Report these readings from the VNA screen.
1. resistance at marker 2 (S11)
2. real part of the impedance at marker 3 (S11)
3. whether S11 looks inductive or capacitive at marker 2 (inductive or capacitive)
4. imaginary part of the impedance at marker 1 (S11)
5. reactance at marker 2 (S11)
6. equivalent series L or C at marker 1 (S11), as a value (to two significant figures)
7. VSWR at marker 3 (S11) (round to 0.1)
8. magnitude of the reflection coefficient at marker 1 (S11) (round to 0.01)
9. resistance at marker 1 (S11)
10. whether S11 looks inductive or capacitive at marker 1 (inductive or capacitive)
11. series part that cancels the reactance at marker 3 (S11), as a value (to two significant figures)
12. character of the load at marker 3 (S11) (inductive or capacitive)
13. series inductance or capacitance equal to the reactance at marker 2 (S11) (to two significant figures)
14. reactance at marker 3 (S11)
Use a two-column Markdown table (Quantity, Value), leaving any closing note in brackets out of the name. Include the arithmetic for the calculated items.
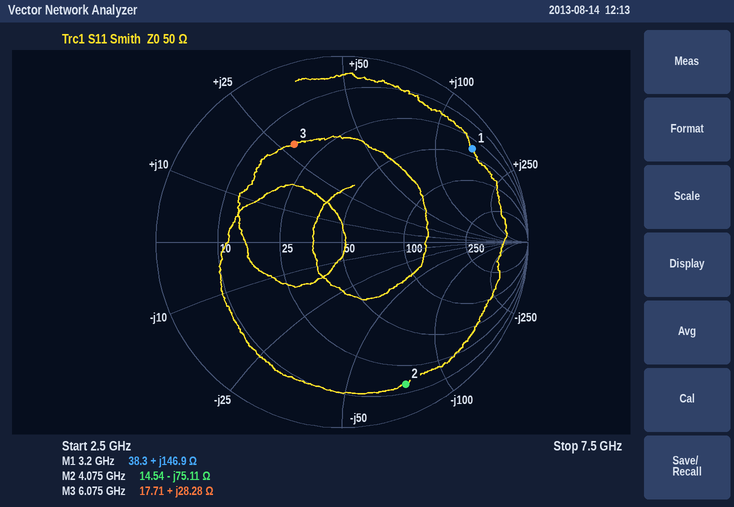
| Quantity | Value |
|---|---|
| resistance at marker 2 | 14.54 Ω |
| real part of the impedance at marker 3 | 17.71 Ω |
| whether S11 looks inductive or capacitive at marker 2 | capacitive |
| imaginary part of the impedance at marker 1 | +146.9 Ω |
| reactance at marker 2 | -75.11 Ω |
| equivalent series L or C at marker 1 (S11), as a value | L = 146.9 Ω/(2π × 3.2 GHz) ≈ 7.3 nH |
| VSWR at marker 3 (S11) | 3.8 |
| magnitude of the reflection coefficient at marker 1 (S11) | 0.86 |
| resistance at marker 1 | 38.3 Ω |
| whether S11 looks inductive or capacitive at marker 1 | inductive |
| series part that cancels the reactance at marker 3 (S11), as a value | C = 1/(2π × 6.075 GHz × 28.28 Ω) ≈ 926 fF, so 930 fF to two significant figures |
| character of the load at marker 3 (S11) | inductive |
| series inductance or capacitance equal to the reactance at marker 2 (S11) | C = 1/(2π × 4.075 GHz × 75.11 Ω) ≈ 520 fF |
| reactance at marker 3 | +28.28 Ω |
